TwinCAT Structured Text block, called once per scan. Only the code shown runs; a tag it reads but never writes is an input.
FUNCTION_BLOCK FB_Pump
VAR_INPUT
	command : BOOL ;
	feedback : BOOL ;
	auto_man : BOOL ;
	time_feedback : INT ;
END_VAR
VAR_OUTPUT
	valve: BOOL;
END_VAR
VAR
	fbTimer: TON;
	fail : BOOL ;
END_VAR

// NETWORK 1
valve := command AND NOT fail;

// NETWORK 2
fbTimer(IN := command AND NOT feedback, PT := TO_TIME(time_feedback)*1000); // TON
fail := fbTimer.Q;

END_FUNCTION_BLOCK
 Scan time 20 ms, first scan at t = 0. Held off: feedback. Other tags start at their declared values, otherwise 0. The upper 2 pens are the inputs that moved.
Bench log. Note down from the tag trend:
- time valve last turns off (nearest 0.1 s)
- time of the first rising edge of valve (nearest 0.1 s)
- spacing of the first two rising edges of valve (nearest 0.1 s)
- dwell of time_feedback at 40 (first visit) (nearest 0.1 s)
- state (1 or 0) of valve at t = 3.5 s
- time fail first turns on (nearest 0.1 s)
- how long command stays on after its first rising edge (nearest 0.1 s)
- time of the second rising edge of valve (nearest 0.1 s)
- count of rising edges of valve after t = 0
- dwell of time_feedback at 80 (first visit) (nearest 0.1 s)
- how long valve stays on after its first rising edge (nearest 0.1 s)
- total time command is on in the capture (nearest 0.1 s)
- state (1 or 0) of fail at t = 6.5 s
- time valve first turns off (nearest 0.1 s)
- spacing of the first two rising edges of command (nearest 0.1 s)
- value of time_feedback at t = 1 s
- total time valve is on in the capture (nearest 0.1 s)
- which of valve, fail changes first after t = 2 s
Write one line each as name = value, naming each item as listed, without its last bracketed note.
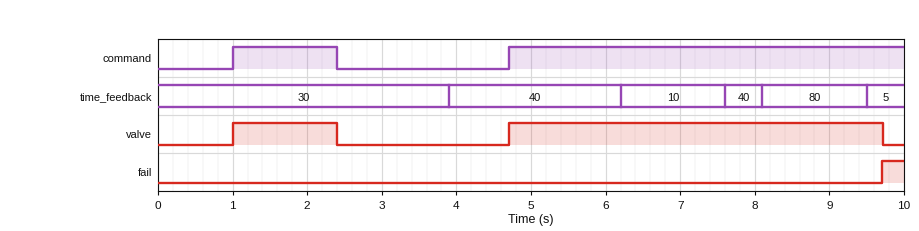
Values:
time valve last turns off = 9.7 s
time of the first rising edge of valve = 1.0 s
spacing of the first two rising edges of valve = 3.7 s
dwell of time_feedback at 40 (first visit) = 2.3 s
state (1 or 0) of valve at t = 3.5 s = 0
time fail first turns on = 9.7 s
how long command stays on after its first rising edge = 1.4 s
time of the second rising edge of valve = 4.7 s
count of rising edges of valve after t = 0 = 2
dwell of time_feedback at 80 (first visit) = 1.4 s
how long valve stays on after its first rising edge = 1.4 s
total time command is on in the capture = 6.7 s
state (1 or 0) of fail at t = 6.5 s = 0
time valve first turns off = 2.4 s
spacing of the first two rising edges of command = 3.7 s
value of time_feedback at t = 1 s = 30
total time valve is on in the capture = 6.4 s
which of valve, fail changes first after t = 2 s = valve
